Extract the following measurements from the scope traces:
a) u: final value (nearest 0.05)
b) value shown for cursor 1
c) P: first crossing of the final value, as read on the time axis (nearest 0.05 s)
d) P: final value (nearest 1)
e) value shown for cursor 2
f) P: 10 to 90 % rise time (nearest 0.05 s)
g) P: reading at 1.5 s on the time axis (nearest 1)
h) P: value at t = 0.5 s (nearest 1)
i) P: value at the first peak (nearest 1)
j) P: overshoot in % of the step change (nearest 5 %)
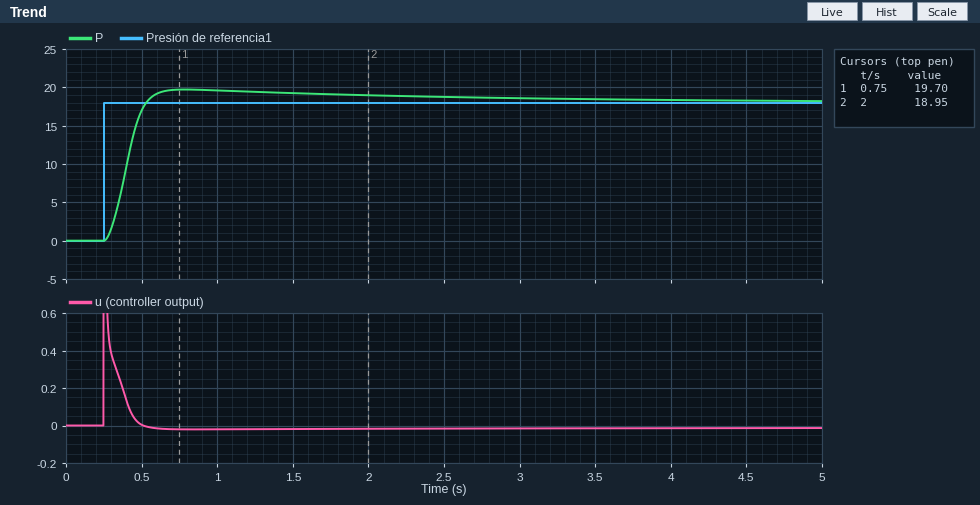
0.00
19.70
0.55 s
18
18.95
0.20 s
19
17
20
10 %
